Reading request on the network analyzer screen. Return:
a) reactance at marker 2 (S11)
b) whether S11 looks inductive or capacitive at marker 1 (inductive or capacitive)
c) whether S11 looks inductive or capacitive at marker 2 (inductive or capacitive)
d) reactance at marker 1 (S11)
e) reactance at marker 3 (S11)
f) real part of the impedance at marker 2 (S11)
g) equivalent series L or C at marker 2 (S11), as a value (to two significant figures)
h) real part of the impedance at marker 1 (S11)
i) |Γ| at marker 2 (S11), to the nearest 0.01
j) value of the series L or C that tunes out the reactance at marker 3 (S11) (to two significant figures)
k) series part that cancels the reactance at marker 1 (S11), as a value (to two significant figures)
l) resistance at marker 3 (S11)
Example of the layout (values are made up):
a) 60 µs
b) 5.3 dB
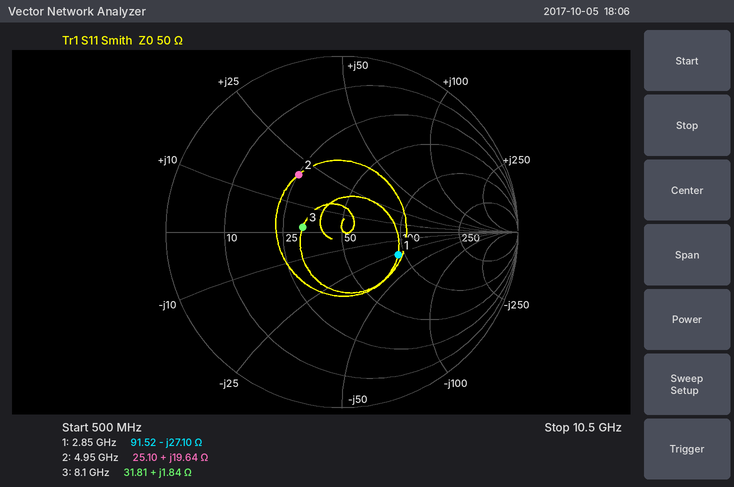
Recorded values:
a) +19.64 Ω
b) capacitive
c) inductive
d) -27.10 Ω
e) +1.84 Ω
f) 25.10 Ω
g) 630 pH
h) 91.52 Ω
i) 0.41
j) 11 pF
k) 1.5 nH
l) 31.81 Ω
